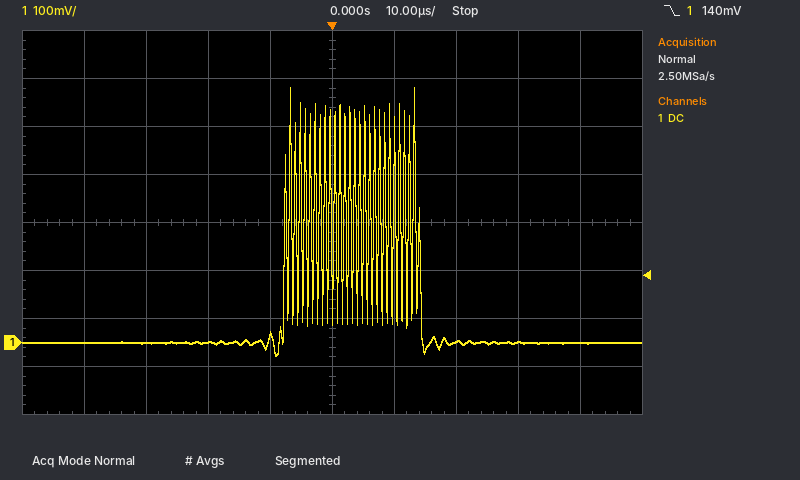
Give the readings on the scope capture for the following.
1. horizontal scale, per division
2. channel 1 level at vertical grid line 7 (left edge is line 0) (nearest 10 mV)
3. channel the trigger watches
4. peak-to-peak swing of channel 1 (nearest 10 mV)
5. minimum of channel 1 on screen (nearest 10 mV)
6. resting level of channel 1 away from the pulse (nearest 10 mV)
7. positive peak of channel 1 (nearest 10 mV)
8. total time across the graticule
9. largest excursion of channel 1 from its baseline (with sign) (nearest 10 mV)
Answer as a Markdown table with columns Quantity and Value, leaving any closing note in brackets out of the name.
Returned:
| Quantity | Value |
|---|---|
| horizontal scale, per division | 10 µs |
| channel 1 level at vertical grid line 7 (left edge is line 0) | 0 mV |
| channel the trigger watches | channel 1 |
| peak-to-peak swing of channel 1 | 560 mV |
| minimum of channel 1 on screen | -30 mV |
| resting level of channel 1 away from the pulse | 0 mV |
| positive peak of channel 1 | 530 mV |
| total time across the graticule | 100 µs |
| largest excursion of channel 1 from its baseline (with sign) | +530 mV |
